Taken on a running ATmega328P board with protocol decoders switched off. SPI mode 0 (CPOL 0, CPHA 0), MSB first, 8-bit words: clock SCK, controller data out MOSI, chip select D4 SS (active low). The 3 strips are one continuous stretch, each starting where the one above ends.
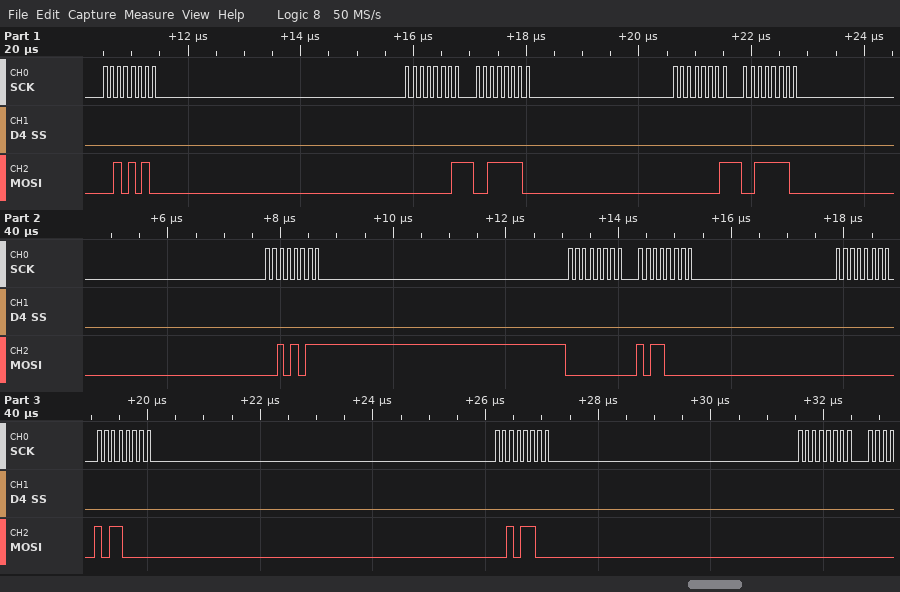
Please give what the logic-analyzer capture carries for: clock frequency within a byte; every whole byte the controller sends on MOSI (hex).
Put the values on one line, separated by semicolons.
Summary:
8 MHz; 2A 01 3E 01 3E 2B 00 B0 00 B0 2C 00
